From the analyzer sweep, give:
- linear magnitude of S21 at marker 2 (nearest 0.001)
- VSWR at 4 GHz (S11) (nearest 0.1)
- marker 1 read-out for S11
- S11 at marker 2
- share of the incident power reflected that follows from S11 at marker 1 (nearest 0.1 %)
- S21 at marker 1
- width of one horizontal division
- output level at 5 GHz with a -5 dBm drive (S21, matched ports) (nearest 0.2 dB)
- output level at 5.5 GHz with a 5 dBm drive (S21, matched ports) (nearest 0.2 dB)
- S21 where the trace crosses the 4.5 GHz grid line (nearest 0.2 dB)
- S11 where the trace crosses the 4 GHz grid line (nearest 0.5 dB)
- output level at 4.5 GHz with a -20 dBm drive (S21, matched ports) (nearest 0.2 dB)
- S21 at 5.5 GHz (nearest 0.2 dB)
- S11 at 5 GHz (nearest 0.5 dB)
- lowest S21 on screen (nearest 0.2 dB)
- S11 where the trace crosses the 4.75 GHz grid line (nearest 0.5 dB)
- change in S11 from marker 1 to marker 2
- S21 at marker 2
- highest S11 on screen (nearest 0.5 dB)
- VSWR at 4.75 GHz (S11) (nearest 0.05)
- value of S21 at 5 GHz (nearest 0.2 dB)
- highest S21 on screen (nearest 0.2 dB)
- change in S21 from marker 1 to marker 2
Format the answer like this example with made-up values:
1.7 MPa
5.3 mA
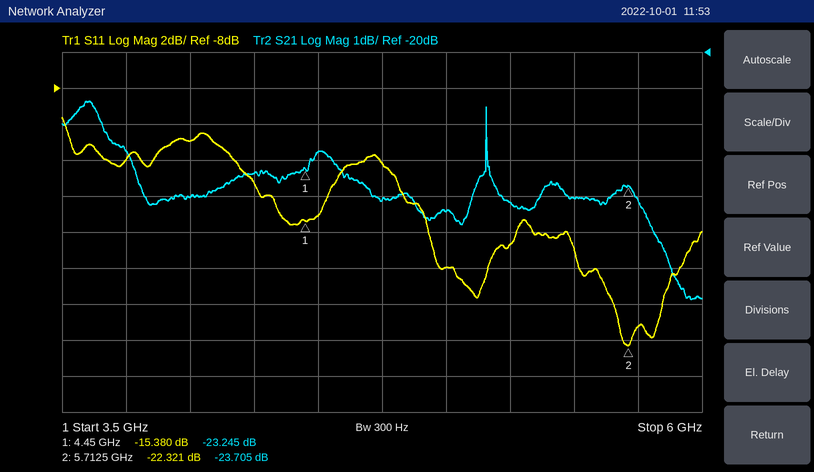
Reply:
0.065
1.8
-15.380 dB
-22.321 dB
2.9 %
-23.245 dB
250 MHz
-29.4 dBm
-19.0 dBm
-22.8 dB
-11.0 dB
-42.8 dBm
-24.0 dB
-18.0 dB
-26.8 dB
-12.0 dB
-6.941 dB
-23.705 dB
-9.5 dB
1.65
-24.4 dB
-21.4 dB
-0.460 dB
